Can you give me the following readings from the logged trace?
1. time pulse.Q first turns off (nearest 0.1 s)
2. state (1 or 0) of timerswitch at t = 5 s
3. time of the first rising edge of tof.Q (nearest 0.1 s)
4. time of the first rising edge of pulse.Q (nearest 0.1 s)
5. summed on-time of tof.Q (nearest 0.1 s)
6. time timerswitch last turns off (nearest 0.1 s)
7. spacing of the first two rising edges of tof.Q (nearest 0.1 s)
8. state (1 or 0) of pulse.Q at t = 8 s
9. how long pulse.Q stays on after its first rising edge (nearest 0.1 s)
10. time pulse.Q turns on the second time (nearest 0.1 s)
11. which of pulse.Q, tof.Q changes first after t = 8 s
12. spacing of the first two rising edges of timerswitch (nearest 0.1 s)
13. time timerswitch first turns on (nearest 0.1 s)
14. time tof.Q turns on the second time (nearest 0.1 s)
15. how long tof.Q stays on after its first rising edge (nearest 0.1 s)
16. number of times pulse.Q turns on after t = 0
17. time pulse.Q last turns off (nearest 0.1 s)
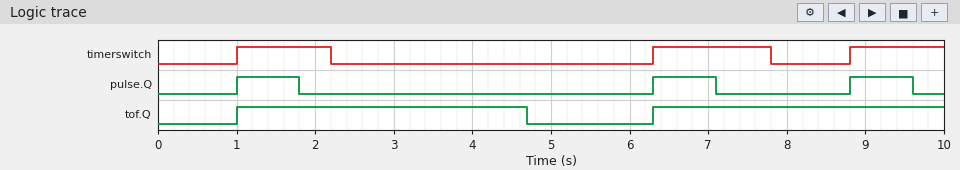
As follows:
1.8 s
0
1.0 s
1.0 s
7.4 s
7.8 s
5.3 s
0
0.8 s
6.3 s
pulse.Q
5.3 s
1.0 s
6.3 s
3.7 s
3
9.6 s
